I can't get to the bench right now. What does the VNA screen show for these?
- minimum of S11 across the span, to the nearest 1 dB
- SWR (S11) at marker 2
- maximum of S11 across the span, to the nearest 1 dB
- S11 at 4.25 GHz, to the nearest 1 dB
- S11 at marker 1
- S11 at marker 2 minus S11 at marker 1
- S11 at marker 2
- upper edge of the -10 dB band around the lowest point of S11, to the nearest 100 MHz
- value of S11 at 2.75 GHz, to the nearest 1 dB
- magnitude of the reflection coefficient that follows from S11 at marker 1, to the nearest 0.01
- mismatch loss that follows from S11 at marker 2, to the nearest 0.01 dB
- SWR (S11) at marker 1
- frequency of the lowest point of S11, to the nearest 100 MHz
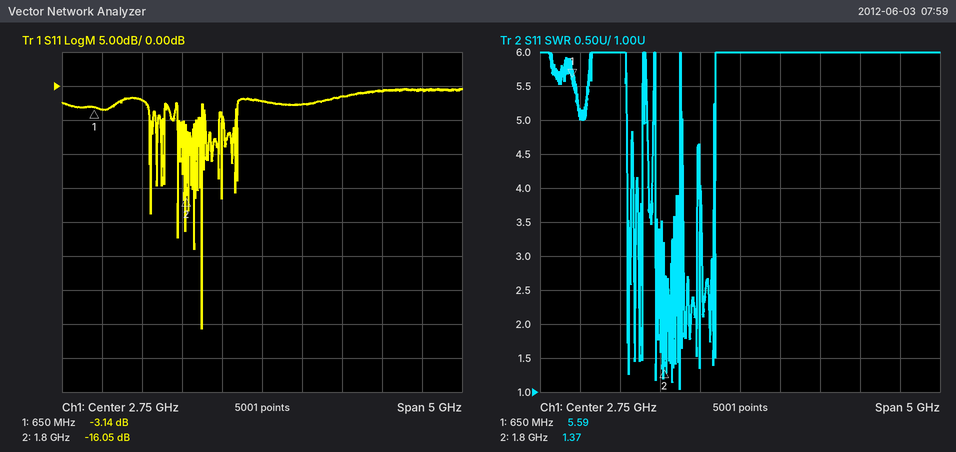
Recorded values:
-36 dB
1.37
0 dB
-1 dB
-3.14 dB
-12.91 dB
-16.05 dB
2.0 GHz
-2 dB
0.70
0.11 dB
5.59
2.0 GHz
